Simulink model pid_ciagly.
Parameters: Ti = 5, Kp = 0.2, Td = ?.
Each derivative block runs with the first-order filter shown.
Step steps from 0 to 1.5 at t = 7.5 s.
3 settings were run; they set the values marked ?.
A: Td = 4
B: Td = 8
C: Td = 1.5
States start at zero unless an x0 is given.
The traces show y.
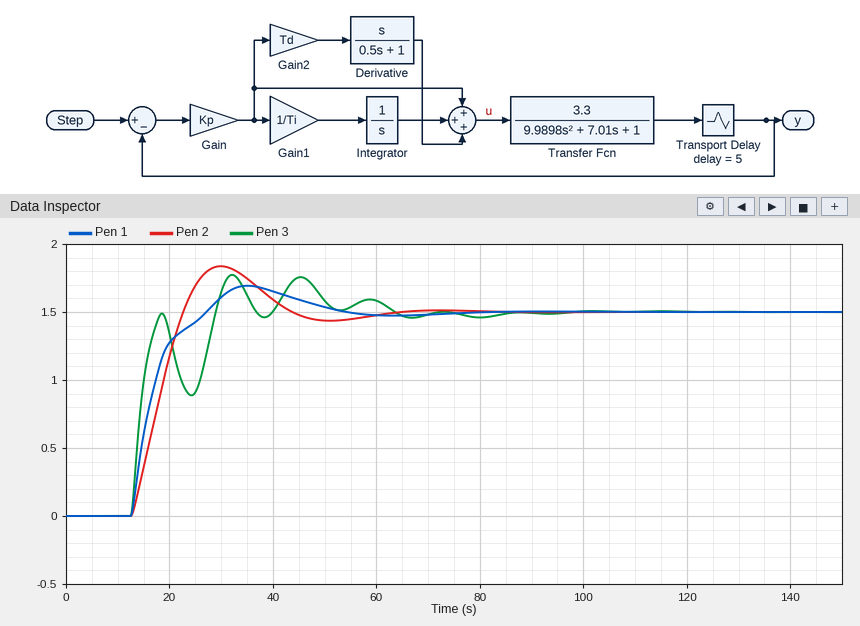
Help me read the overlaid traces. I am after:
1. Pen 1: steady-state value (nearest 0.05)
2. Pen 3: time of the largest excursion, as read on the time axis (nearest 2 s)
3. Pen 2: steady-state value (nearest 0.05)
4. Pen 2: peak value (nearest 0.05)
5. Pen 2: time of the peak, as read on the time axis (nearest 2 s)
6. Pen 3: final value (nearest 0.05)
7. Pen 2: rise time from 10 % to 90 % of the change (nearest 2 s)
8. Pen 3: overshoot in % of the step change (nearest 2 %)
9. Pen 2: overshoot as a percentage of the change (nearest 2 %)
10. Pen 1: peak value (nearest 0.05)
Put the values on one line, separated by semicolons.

1.50; 32 s; 1.50; 1.85; 30 s; 1.50; 8 s; 18 %; 22 %; 1.70
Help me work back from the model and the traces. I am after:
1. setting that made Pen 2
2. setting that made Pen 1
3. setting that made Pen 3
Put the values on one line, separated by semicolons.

C; A; B
